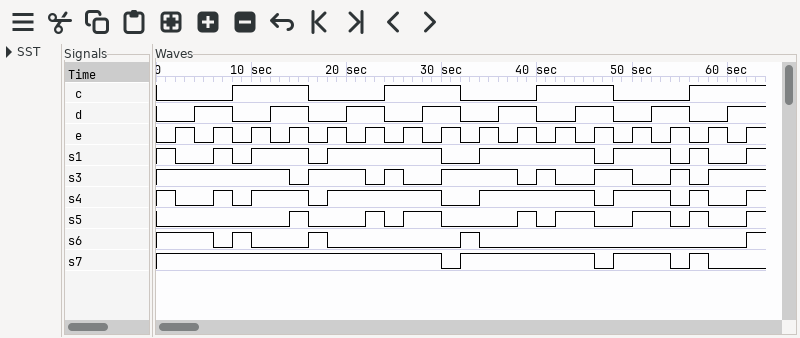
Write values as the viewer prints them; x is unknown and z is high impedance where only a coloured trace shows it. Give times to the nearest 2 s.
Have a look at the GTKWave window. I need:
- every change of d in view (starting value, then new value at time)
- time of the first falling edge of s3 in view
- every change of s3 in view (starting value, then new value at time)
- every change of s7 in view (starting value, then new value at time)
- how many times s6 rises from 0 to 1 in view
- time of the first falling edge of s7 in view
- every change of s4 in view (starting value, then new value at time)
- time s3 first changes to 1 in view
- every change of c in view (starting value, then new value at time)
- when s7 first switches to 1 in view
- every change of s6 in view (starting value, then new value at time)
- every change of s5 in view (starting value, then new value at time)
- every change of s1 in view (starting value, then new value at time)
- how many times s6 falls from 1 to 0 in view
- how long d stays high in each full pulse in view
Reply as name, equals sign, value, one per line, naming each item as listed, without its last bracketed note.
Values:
every change of d in view = 0, 1 at 4 s, 0 at 8 s, 1 at 12 s, 0 at 16 s, 1 at 20 s, 0 at 24 s, 1 at 28 s, 0 at 32 s, 1 at 36 s, 0 at 40 s, 1 at 44 s, 0 at 48 s, 1 at 52 s, 0 at 56 s, 1 at 60 s
time of the first falling edge of s3 in view = 14 s
every change of s3 in view = 1, 0 at 14 s, 1 at 16 s, 0 at 22 s, 1 at 24 s, 0 at 26 s, 1 at 30 s, 0 at 38 s, 1 at 40 s, 0 at 42 s, 1 at 46 s, 0 at 50 s, 1 at 54 s, 0 at 56 s, 1 at 58 s
every change of s7 in view = 1, 0 at 30 s, 1 at 32 s, 0 at 46 s, 1 at 48 s, 0 at 54 s, 1 at 56 s, 0 at 58 s
how many times s6 rises from 0 to 1 in view = 4
time of the first falling edge of s7 in view = 30 s
every change of s4 in view = 1, 0 at 2 s, 1 at 6 s, 0 at 8 s, 1 at 10 s, 0 at 16 s, 1 at 18 s, 0 at 30 s, 1 at 34 s, 0 at 46 s, 1 at 48 s, 0 at 54 s, 1 at 56 s, 0 at 58 s, 1 at 62 s
time s3 first changes to 1 in view = 16 s
every change of c in view = 0, 1 at 8 s, 0 at 16 s, 1 at 24 s, 0 at 32 s, 1 at 40 s, 0 at 48 s, 1 at 56 s
when s7 first switches to 1 in view = 32 s
every change of s6 in view = 1, 0 at 6 s, 1 at 8 s, 0 at 10 s, 1 at 16 s, 0 at 18 s, 1 at 32 s, 0 at 34 s, 1 at 62 s
every change of s5 in view = 0, 1 at 14 s, 0 at 16 s, 1 at 22 s, 0 at 24 s, 1 at 26 s, 0 at 30 s, 1 at 38 s, 0 at 40 s, 1 at 42 s, 0 at 46 s, 1 at 50 s, 0 at 54 s, 1 at 56 s, 0 at 58 s, 1 at 62 s
every change of s1 in view = 1, 0 at 2 s, 1 at 6 s, 0 at 8 s, 1 at 10 s, 0 at 16 s, 1 at 18 s, 0 at 30 s, 1 at 34 s, 0 at 46 s, 1 at 48 s, 0 at 54 s, 1 at 56 s, 0 at 58 s, 1 at 62 s
how many times s6 falls from 1 to 0 in view = 4
how long d stays high in each full pulse in view = 4 s, 4 s, 4 s, 4 s, 4 s, 4 s, 4 s
